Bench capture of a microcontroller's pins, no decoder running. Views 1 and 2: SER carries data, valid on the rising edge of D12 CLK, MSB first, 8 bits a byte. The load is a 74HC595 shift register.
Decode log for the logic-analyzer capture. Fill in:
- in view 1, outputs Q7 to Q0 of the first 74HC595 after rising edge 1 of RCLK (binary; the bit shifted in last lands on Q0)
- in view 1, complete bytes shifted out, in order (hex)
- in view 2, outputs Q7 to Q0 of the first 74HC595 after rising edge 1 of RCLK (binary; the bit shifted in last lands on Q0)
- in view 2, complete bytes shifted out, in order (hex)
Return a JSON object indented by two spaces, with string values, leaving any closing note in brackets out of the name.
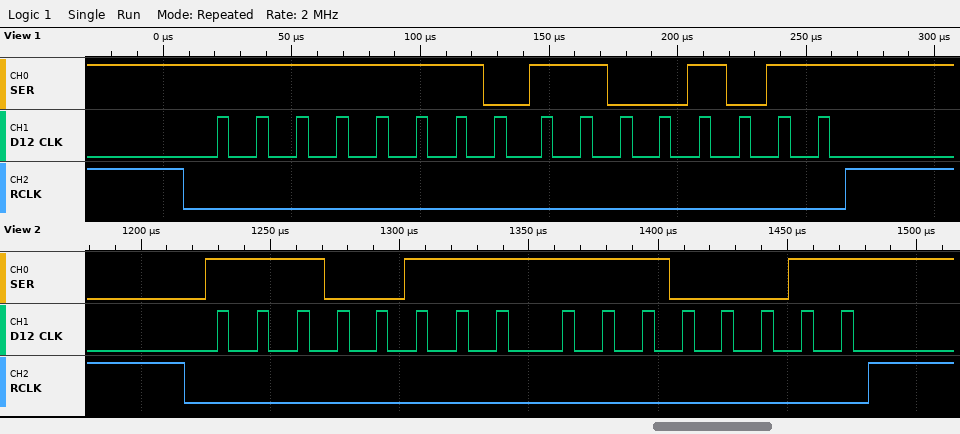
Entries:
{
  "in view 1, outputs Q7 to Q0 of the first 74HC595 after rising edge 1 of RCLK": "11001011",
  "in view 1, complete bytes shifted out, in order": "FE CB",
  "in view 2, outputs Q7 to Q0 of the first 74HC595 after rising edge 1 of RCLK": "11100011",
  "in view 2, complete bytes shifted out, in order": "0xE7 0xE3"
}
